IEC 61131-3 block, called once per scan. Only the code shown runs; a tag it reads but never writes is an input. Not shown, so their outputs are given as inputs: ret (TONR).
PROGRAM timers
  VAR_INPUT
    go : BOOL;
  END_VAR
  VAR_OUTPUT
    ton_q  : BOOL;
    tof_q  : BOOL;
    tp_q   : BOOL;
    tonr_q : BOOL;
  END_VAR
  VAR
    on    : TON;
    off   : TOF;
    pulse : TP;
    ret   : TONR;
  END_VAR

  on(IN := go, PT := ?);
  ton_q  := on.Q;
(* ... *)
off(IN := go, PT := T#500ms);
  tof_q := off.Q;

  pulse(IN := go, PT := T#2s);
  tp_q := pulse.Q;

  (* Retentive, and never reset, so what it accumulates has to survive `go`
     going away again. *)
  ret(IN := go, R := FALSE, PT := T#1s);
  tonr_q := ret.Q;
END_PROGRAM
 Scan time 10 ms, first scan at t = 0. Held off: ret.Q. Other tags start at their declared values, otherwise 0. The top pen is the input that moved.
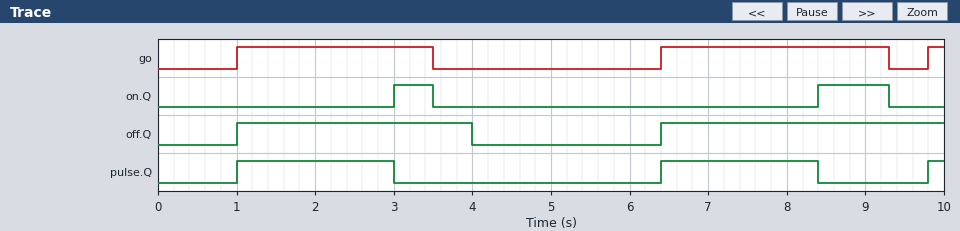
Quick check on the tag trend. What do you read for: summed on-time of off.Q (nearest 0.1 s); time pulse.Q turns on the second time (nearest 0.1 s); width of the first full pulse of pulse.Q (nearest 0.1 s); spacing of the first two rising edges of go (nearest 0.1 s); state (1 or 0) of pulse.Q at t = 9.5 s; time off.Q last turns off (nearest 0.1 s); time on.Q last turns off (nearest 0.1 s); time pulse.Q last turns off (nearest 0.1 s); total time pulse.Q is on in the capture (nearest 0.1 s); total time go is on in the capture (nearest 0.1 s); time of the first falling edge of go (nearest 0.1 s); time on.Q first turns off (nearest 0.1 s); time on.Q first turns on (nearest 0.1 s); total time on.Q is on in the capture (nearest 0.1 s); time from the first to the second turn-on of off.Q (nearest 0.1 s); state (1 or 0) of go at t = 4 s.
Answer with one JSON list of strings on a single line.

["6.6 s", "6.4 s", "2.0 s", "5.4 s", "0", "4.0 s", "9.3 s", "8.4 s", "4.2 s", "5.6 s", "3.5 s", "3.5 s", "3.0 s", "1.4 s", "5.4 s", "0"]
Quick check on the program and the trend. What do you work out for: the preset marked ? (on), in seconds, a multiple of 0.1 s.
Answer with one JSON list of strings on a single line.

["2.0 s"]
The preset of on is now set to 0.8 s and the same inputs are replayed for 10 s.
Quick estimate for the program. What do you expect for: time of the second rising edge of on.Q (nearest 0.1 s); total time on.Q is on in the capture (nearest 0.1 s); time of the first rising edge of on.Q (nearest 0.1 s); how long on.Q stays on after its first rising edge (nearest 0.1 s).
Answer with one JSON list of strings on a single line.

["7.2 s", "3.8 s", "1.8 s", "1.7 s"]
